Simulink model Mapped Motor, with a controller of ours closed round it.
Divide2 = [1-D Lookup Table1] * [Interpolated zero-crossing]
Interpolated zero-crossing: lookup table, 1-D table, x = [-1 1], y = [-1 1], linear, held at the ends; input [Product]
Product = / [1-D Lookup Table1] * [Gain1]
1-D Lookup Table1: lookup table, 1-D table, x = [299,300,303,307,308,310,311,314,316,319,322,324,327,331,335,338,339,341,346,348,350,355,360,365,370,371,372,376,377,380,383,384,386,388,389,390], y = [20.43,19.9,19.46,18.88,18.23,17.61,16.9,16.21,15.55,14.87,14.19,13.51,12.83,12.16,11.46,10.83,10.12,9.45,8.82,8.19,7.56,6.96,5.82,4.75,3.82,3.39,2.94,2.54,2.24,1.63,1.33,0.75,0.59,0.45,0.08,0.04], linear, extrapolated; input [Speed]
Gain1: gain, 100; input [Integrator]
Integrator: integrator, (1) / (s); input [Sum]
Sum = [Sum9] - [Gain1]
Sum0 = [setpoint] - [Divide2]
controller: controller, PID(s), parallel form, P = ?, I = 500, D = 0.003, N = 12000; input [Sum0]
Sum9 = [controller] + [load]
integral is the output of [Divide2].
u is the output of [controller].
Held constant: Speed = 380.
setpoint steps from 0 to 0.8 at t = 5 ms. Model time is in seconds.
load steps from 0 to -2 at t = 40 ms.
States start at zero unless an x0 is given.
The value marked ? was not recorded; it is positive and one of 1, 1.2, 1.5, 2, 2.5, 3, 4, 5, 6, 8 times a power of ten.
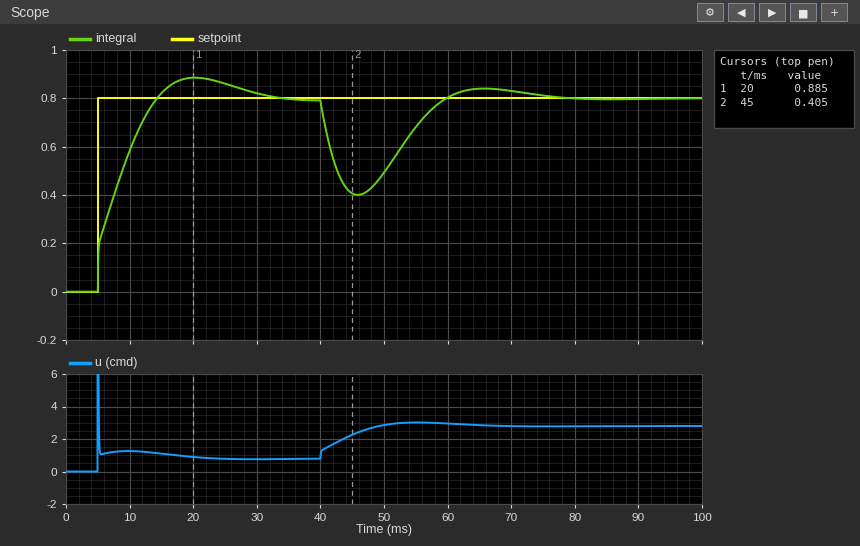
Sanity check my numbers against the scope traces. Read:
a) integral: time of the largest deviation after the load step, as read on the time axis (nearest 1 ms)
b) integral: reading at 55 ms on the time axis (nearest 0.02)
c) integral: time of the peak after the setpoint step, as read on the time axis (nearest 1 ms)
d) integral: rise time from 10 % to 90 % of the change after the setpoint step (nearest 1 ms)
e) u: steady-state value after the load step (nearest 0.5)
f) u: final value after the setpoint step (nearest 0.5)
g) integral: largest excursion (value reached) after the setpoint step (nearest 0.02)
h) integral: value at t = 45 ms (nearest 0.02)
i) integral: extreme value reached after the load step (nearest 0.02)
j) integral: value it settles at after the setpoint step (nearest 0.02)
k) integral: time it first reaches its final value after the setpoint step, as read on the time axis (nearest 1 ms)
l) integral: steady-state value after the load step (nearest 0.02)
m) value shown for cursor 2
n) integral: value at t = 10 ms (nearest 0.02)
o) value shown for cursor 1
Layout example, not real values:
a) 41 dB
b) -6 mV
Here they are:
a) 46 ms
b) 0.68
c) 20 ms
d) 7 ms
e) 3.0
f) 1.0
g) 0.88
h) 0.40
i) 0.40
j) 0.80
k) 14 ms
l) 0.80
m) 0.405
n) 0.58
o) 0.885
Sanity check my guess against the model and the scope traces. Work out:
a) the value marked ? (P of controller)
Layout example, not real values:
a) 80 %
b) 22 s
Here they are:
a) 2
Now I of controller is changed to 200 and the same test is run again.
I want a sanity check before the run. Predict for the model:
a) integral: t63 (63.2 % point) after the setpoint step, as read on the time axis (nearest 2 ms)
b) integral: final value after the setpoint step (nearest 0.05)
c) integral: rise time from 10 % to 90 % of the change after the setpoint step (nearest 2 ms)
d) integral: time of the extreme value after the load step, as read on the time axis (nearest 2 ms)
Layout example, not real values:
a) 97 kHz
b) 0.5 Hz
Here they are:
a) 10 ms
b) 0.80
c) 14 ms
d) 48 ms
